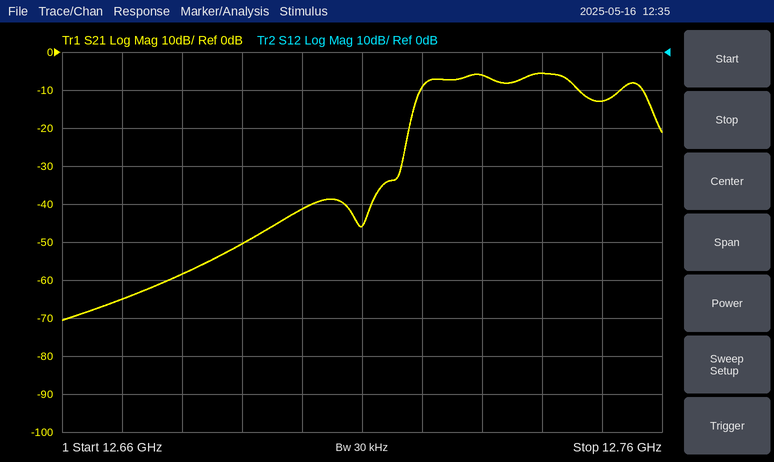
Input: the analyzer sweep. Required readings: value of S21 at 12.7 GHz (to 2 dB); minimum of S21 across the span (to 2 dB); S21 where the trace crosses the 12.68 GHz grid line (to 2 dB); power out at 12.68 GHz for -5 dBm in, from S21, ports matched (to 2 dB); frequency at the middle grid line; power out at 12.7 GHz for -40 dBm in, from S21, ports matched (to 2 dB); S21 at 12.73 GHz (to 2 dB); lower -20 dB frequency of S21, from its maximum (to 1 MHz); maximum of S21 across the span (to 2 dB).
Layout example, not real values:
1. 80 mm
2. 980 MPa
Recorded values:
1. -42 dB
2. -70 dB
3. -58 dB
4. -64 dBm
5. 12.71 GHz
6. -82 dBm
7. -6 dB
8. 12.717 GHz
9. -6 dB
